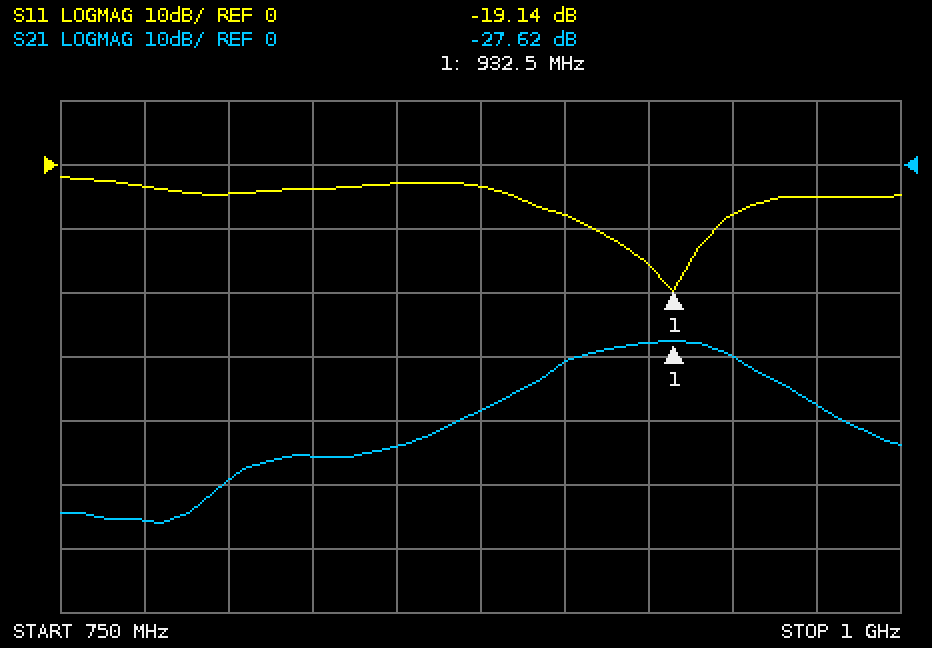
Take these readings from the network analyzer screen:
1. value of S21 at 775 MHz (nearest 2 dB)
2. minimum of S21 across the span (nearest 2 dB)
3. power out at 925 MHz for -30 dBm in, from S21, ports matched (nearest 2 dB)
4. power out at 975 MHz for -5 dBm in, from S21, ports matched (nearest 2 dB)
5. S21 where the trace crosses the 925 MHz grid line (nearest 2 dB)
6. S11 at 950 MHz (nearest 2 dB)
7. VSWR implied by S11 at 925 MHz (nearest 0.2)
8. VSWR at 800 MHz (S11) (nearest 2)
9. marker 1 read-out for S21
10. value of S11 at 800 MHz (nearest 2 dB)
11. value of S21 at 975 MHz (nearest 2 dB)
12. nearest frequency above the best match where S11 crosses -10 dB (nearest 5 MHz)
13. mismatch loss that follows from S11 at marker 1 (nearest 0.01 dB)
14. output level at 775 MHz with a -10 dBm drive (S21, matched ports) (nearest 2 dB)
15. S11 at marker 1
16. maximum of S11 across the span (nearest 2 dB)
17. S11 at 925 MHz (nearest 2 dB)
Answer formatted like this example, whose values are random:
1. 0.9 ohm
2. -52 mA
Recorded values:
1. -56 dB
2. -56 dB
3. -58 dBm
4. -42 dBm
5. -28 dB
6. -8 dB
7. 1.4
8. 4
9. -27.62 dB
10. -4 dB
11. -38 dB
12. 945 MHz
13. 0.05 dB
14. -66 dBm
15. -19.14 dB
16. -2 dB
17. -16 dB
